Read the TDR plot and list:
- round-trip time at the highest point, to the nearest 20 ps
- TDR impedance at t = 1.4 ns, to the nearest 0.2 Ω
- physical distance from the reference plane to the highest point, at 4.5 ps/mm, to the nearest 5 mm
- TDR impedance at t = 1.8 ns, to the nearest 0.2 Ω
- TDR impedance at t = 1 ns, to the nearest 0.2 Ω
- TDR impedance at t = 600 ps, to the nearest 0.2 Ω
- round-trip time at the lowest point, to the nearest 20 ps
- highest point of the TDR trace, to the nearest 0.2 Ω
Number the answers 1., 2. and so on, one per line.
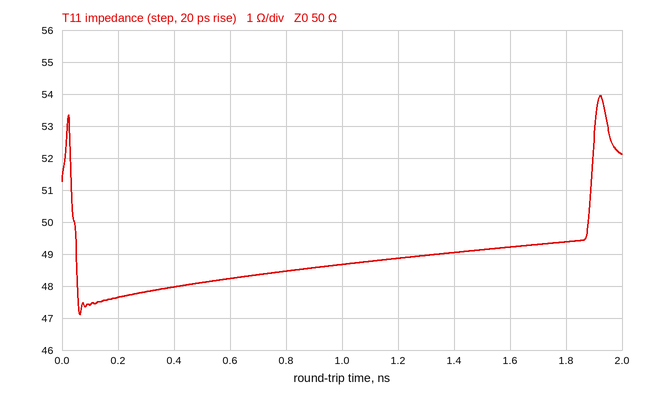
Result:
1. 1.92 ns
2. 49.0 Ω
3. 215 mm
4. 49.4 Ω
5. 48.6 Ω
6. 48.2 Ω
7. 60 ps
8. 54.0 Ω
